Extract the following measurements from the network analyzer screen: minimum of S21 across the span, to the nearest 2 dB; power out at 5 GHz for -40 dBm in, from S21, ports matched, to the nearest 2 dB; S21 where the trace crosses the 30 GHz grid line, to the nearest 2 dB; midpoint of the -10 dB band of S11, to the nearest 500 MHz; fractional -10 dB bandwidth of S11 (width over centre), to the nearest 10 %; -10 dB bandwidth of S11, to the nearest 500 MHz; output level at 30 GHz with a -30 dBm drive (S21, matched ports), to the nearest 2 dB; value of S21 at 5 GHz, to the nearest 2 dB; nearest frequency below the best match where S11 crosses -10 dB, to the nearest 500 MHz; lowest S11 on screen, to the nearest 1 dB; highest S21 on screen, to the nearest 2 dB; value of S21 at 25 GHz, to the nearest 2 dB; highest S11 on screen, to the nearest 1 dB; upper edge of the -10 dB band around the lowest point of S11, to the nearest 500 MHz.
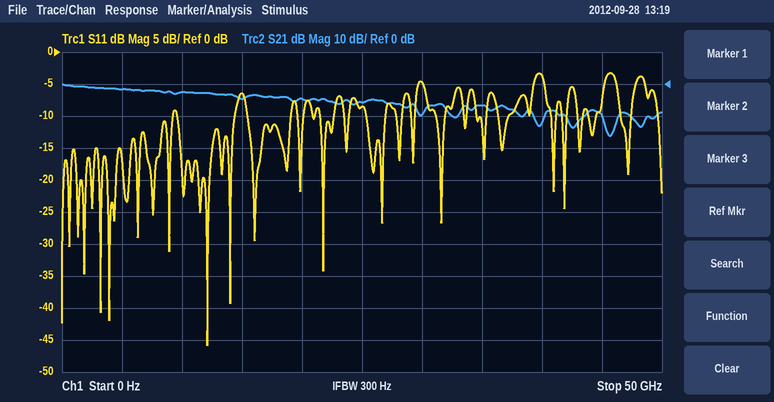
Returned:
-16 dB
-42 dBm
-10 dB
12.0 GHz
40 %
5.0 GHz
-40 dBm
-2 dB
9.5 GHz
-46 dB
0 dB
-6 dB
-3 dB
14.5 GHz
